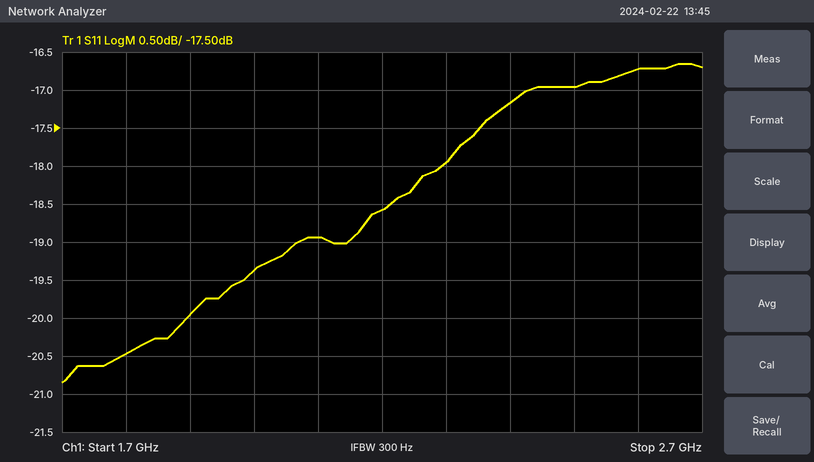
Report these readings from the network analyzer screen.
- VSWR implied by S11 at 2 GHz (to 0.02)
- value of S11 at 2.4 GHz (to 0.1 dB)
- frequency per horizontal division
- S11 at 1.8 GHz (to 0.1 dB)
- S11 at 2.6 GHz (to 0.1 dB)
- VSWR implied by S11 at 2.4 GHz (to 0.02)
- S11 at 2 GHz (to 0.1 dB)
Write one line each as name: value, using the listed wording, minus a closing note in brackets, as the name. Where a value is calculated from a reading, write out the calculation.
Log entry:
VSWR implied by S11 at 2 GHz: |Γ| = 10^(-19.4/20) = 0.1072; VSWR = (1 + 0.1072)/(1 − 0.1072) ≈ 1.24
value of S11 at 2.4 GHz: -17.2 dB
frequency per horizontal division: 100 MHz
S11 at 1.8 GHz: -20.5 dB
S11 at 2.6 GHz: -16.7 dB
VSWR implied by S11 at 2.4 GHz: |Γ| = 10^(-17.2/20) = 0.1380; VSWR = (1 + 0.1380)/(1 − 0.1380) ≈ 1.32
S11 at 2 GHz: -19.4 dB
